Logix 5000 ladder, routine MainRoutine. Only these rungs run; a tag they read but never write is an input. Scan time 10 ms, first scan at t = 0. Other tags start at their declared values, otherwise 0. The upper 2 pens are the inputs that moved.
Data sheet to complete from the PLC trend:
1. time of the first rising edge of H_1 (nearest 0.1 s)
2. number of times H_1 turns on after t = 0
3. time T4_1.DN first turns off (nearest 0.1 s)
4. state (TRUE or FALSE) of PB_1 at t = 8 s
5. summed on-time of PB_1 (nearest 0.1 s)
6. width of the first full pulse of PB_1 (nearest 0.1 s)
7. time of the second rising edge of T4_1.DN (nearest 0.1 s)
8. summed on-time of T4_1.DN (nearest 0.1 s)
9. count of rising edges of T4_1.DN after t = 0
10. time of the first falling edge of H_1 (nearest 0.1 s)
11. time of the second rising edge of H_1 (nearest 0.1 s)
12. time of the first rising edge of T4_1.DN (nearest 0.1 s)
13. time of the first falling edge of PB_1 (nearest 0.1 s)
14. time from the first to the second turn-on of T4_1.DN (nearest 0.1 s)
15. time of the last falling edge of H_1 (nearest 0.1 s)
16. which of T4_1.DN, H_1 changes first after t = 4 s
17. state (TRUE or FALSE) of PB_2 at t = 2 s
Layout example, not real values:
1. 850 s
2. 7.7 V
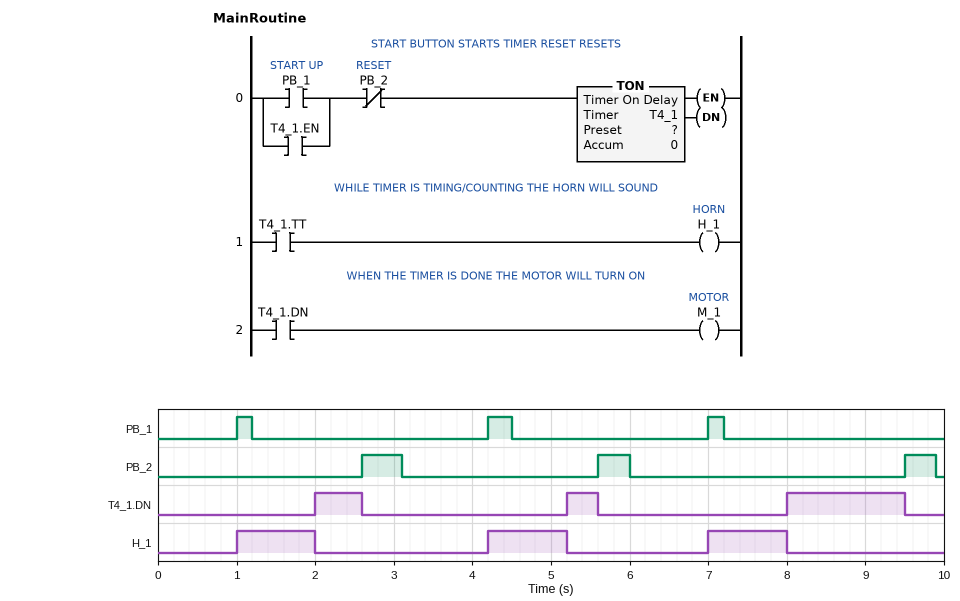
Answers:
1. 1.0 s
2. 3
3. 2.6 s
4. FALSE
5. 0.7 s
6. 0.2 s
7. 5.2 s
8. 2.5 s
9. 3
10. 2.0 s
11. 4.2 s
12. 2.0 s
13. 1.2 s
14. 3.2 s
15. 8.0 s
16. H_1
17. FALSE
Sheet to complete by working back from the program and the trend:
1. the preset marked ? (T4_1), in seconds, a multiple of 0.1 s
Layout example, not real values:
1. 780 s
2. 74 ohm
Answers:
1. 1.0 s
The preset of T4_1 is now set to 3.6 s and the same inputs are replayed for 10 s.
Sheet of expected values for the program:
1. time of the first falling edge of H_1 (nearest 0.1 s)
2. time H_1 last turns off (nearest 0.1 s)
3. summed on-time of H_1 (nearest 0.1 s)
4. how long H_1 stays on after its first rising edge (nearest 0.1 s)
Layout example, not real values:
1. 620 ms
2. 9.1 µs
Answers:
1. 2.6 s
2. 9.5 s
3. 5.5 s
4. 1.6 s
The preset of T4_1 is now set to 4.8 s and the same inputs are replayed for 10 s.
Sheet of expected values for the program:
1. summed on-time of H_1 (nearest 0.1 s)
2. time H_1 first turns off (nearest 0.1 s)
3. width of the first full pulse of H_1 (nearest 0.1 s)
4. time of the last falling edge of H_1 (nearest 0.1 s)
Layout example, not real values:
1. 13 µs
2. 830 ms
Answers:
1. 5.5 s
2. 2.6 s
3. 1.6 s
4. 9.5 s
